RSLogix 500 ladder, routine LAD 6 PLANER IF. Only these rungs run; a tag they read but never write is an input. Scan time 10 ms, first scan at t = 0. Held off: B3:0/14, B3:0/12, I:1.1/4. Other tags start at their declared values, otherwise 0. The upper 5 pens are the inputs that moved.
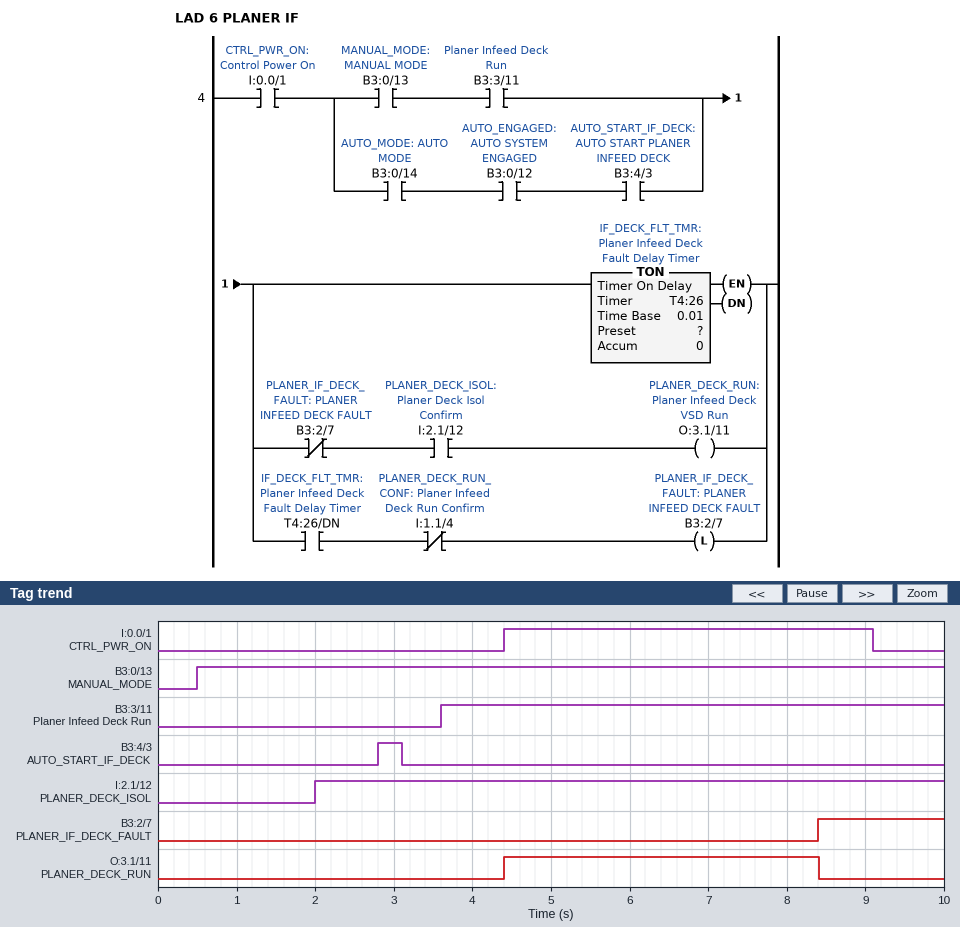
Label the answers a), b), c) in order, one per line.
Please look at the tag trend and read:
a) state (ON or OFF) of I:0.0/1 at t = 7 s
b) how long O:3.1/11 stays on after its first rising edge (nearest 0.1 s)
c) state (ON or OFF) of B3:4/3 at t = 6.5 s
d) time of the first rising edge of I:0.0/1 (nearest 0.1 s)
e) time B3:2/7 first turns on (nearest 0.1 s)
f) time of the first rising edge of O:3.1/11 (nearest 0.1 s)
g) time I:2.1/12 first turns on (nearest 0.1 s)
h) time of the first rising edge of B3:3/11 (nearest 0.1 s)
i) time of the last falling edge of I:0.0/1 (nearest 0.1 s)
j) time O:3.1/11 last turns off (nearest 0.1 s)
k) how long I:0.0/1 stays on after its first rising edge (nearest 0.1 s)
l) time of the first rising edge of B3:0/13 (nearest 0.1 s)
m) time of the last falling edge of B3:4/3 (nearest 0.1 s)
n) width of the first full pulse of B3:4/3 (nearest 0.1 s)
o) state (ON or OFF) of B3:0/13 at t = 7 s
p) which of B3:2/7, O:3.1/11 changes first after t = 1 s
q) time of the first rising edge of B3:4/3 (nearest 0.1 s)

a) ON
b) 4.0 s
c) OFF
d) 4.4 s
e) 8.4 s
f) 4.4 s
g) 2.0 s
h) 3.6 s
i) 9.1 s
j) 8.4 s
k) 4.7 s
l) 0.5 s
m) 3.1 s
n) 0.3 s
o) ON
p) O:3.1/11
q) 2.8 s
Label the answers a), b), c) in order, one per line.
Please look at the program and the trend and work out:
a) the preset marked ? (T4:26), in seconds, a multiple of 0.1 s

a) 4.0 s
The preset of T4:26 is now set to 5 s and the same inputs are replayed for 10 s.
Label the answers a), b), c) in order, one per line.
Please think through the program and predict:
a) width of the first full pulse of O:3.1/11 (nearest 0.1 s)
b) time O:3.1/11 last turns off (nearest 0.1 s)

a) 4.7 s
b) 9.1 s
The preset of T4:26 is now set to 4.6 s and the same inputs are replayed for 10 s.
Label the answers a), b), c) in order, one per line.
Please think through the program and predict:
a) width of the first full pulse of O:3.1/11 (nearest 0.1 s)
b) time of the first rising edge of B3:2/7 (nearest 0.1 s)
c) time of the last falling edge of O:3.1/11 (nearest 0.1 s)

a) 4.6 s
b) 9.0 s
c) 9.0 s
